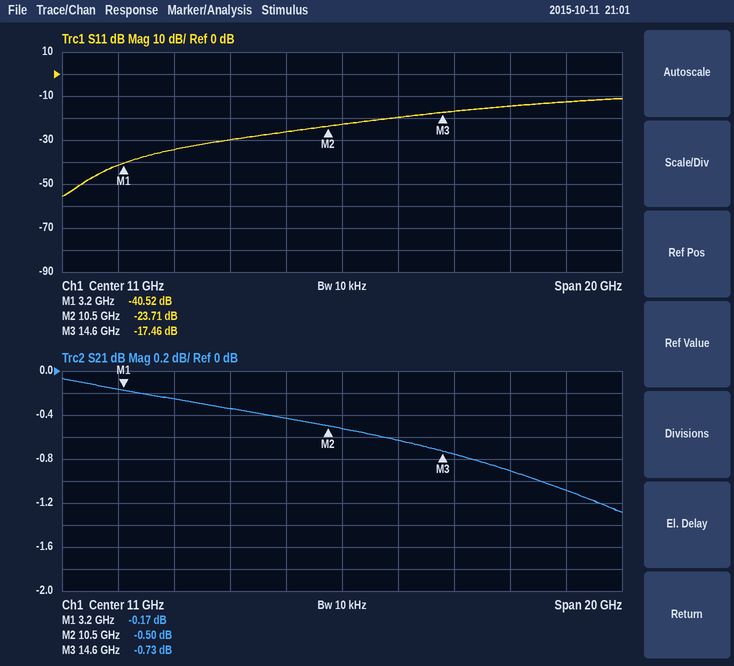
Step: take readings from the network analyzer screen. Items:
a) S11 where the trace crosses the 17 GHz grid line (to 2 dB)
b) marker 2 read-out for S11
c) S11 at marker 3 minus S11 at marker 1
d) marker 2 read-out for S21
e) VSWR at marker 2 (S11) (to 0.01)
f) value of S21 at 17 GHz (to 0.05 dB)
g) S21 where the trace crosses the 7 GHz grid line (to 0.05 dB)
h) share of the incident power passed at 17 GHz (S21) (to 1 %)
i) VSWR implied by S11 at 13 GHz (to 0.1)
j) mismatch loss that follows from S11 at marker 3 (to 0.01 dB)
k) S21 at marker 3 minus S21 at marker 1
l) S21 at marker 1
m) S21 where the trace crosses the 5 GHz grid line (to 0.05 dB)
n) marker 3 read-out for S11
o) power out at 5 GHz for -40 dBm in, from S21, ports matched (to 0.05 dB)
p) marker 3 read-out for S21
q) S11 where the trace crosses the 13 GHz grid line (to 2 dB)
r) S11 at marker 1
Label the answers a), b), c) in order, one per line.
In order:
a) -14 dB
b) -23.71 dB
c) 23.06 dB
d) -0.50 dB
e) 1.14
f) -0.90 dB
g) -0.35 dB
h) 81 %
i) 1.2
j) 0.08 dB
k) -0.56 dB
l) -0.17 dB
m) -0.25 dB
n) -17.46 dB
o) -40.25 dBm
p) -0.73 dB
q) -20 dB
r) -40.52 dB
